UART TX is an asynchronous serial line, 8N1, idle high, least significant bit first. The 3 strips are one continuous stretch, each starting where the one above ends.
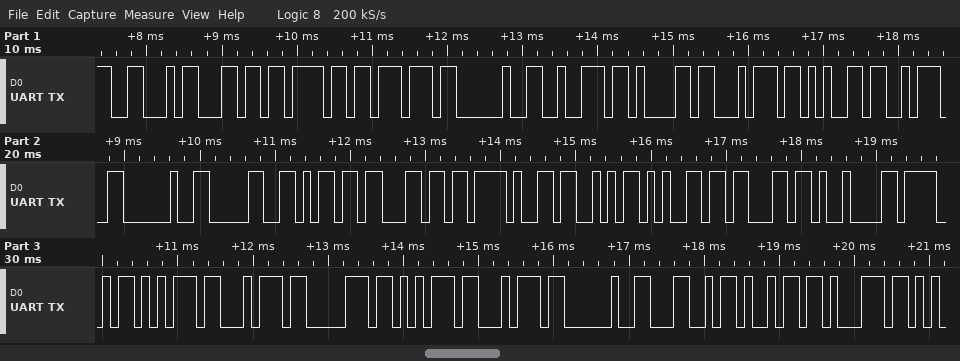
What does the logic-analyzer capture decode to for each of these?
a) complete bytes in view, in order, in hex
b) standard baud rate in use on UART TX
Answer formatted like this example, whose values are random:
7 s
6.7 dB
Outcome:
0x46 0x6C 0x6F 0x77 0x20 0x72 0x61 0x74 0x65 0x3A 0x20 0x30 0x6D 0x6C 0x2F 0x53 0x65 0x63 0x09 0x4F 0x75 0x74 0x70 0x75 0x74 0x20 0x4C 0x69 0x71
9600 baud
